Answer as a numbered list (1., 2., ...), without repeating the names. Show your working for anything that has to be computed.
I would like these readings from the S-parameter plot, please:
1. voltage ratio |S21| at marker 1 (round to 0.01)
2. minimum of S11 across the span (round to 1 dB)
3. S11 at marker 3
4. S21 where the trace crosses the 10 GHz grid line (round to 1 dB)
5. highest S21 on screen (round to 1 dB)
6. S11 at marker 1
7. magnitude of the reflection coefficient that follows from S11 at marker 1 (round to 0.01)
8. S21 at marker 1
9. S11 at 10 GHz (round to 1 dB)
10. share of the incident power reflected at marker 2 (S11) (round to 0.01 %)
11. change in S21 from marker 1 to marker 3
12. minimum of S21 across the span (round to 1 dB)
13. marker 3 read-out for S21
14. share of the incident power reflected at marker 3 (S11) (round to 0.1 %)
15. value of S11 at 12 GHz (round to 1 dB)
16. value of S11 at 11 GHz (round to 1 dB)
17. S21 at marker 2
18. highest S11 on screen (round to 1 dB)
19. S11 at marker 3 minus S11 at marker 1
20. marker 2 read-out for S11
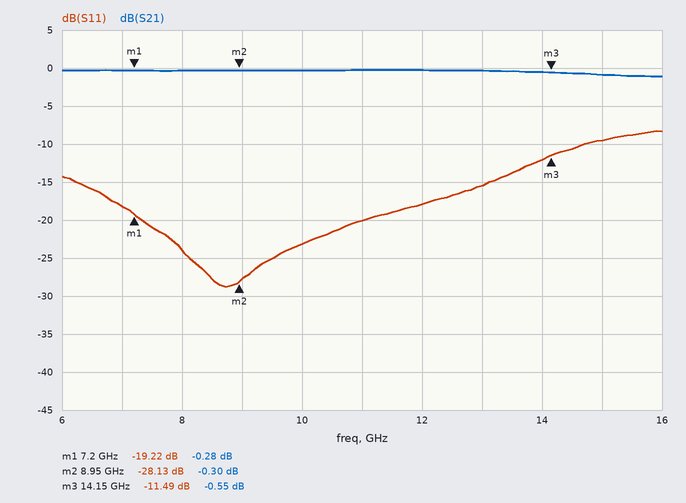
1. 10^(-0.28/20) ≈ 0.97
2. -29 dB
3. -11.49 dB
4. 0 dB
5. 0 dB
6. -19.22 dB
7. 10^(-19.22/20) ≈ 0.11
8. -0.28 dB
9. -23 dB
10. 10^(-28.13/10) ≈ 0.15 %
11. -0.55 − (-0.28) = -0.27 dB
12. -1 dB
13. -0.55 dB
14. 10^(-11.49/10) ≈ 7.1 %
15. -18 dB
16. -20 dB
17. -0.30 dB
18. -8 dB
19. -11.49 − (-19.22) = 7.73 dB
20. -28.13 dB
